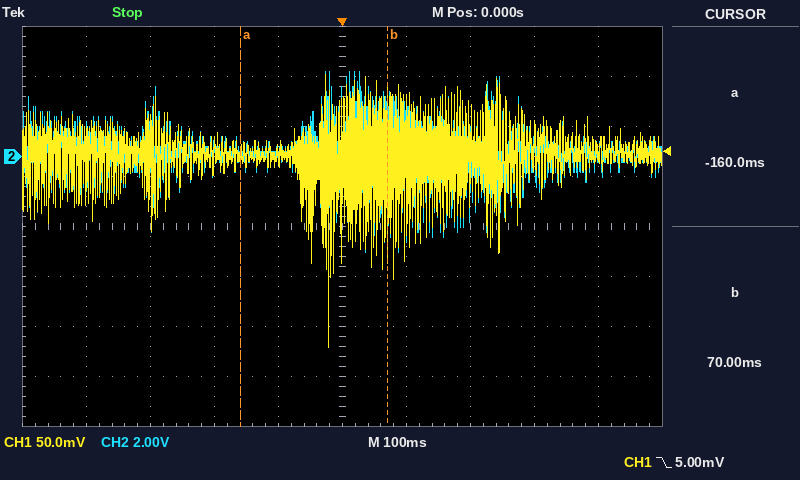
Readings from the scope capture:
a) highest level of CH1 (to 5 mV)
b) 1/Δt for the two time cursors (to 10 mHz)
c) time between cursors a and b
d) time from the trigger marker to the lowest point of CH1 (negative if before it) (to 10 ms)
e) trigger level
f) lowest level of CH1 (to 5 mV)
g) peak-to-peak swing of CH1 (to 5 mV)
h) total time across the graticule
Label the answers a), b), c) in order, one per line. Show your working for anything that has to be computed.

a) 80 mV
b) 1 / 230 ms ≈ 4.35 Hz
c) 70 ms − (-160 ms) = 230 ms
d) -20 ms
e) 5.00 mV
f) -190 mV
g) 80 mV − (-190 mV) = 270 mV
h) 1 s
